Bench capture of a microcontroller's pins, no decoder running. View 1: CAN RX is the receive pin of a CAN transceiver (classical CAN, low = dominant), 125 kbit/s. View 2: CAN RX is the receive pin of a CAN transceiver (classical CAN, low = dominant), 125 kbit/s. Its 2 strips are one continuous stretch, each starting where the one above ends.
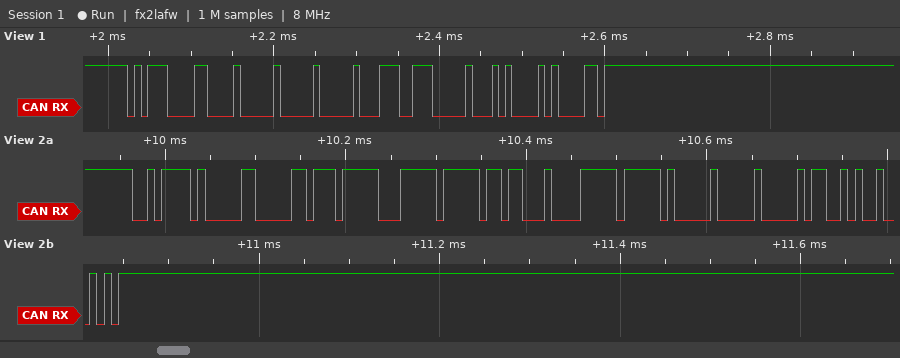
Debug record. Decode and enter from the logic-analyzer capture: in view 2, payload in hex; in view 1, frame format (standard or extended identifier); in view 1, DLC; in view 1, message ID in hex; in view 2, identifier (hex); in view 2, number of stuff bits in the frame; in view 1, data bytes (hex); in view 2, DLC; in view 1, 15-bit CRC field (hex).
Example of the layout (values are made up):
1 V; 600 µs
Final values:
2E F9 FF EC 43 FF 80 00; standard; 4; 0x5C3; 0x2F4; 10; 00 00 E7 00; 8; 0x50A1
